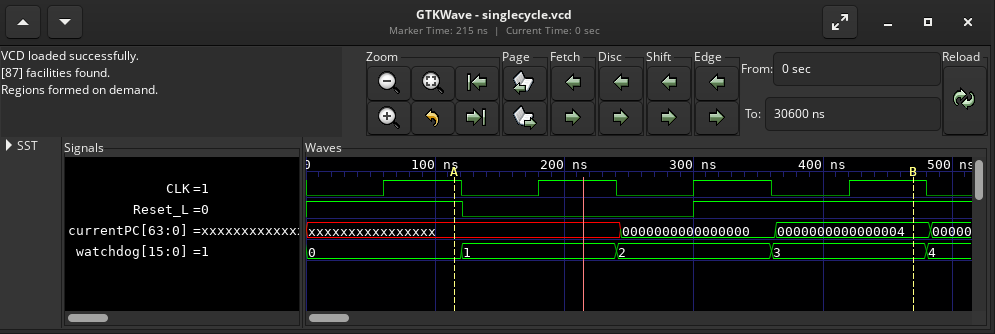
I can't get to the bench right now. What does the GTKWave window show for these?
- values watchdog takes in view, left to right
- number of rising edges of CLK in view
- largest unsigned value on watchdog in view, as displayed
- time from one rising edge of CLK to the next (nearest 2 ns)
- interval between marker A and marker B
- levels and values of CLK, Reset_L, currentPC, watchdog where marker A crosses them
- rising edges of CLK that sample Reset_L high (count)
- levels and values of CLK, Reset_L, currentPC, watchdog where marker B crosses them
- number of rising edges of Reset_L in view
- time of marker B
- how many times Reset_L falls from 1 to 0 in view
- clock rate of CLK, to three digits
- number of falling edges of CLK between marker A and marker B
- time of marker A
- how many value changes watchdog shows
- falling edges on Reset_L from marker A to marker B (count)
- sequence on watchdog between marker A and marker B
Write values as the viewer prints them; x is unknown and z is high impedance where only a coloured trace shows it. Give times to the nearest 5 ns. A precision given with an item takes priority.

0, 1, 2, 3, 4
4
4
120 ns
355 ns
CLK=1, Reset_L=1, currentPC=xxxxxxxxxxxxxxxx, watchdog=0
2
CLK=1, Reset_L=1, currentPC=0000000000000004, watchdog=3
1
470 ns
1
8.33 MHz
3
115 ns
4
1
0, 1, 2, 3
